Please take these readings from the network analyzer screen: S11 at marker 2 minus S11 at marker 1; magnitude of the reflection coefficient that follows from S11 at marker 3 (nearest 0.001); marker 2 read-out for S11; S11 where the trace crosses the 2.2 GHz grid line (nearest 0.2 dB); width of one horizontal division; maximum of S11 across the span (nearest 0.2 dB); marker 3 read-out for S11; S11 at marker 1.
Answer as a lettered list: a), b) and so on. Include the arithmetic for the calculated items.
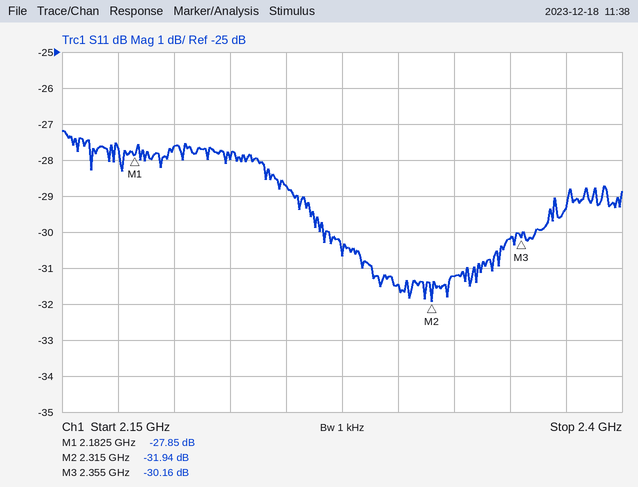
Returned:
a) -31.94 − (-27.85) = -4.09 dB
b) 10^(-30.16/20) ≈ 0.031
c) -31.94 dB
d) -27.6 dB
e) 25 MHz
f) -27.2 dB
g) -30.16 dB
h) -27.85 dB
